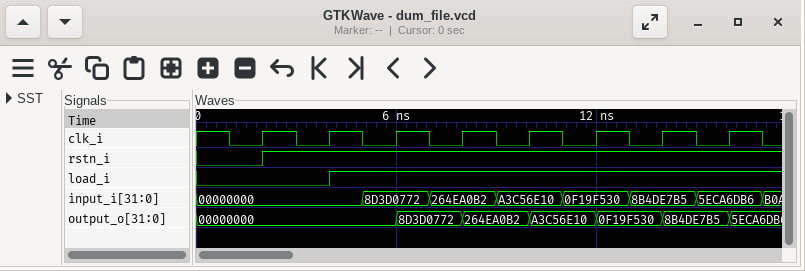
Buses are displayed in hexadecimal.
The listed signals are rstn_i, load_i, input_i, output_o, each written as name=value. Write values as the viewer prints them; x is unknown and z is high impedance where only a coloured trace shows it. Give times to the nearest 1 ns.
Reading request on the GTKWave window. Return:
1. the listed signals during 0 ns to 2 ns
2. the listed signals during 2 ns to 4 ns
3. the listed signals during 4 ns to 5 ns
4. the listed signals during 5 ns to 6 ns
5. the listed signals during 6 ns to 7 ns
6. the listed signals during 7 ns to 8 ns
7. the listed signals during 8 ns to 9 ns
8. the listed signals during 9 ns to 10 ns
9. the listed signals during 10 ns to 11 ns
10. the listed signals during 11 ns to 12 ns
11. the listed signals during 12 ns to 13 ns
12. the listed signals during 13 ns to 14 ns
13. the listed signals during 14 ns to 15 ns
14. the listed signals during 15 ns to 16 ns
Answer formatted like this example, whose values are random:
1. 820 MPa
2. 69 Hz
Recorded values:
1. rstn_i=0, load_i=0, input_i=00000000, output_o=00000000
2. rstn_i=1, load_i=0, input_i=00000000, output_o=00000000
3. rstn_i=1, load_i=1, input_i=00000000, output_o=00000000
4. rstn_i=1, load_i=1, input_i=8D3D0772, output_o=00000000
5. rstn_i=1, load_i=1, input_i=8D3D0772, output_o=8D3D0772
6. rstn_i=1, load_i=1, input_i=264EA0B2, output_o=8D3D0772
7. rstn_i=1, load_i=1, input_i=264EA0B2, output_o=264EA0B2
8. rstn_i=1, load_i=1, input_i=A3C56E10, output_o=264EA0B2
9. rstn_i=1, load_i=1, input_i=A3C56E10, output_o=A3C56E10
10. rstn_i=1, load_i=1, input_i=0F19F530, output_o=A3C56E10
11. rstn_i=1, load_i=1, input_i=0F19F530, output_o=0F19F530
12. rstn_i=1, load_i=1, input_i=8B4DE7B5, output_o=0F19F530
13. rstn_i=1, load_i=1, input_i=8B4DE7B5, output_o=8B4DE7B5
14. rstn_i=1, load_i=1, input_i=5ECA6DB6, output_o=8B4DE7B5
